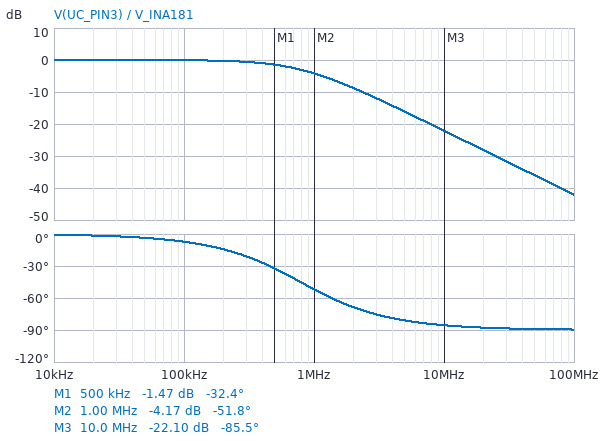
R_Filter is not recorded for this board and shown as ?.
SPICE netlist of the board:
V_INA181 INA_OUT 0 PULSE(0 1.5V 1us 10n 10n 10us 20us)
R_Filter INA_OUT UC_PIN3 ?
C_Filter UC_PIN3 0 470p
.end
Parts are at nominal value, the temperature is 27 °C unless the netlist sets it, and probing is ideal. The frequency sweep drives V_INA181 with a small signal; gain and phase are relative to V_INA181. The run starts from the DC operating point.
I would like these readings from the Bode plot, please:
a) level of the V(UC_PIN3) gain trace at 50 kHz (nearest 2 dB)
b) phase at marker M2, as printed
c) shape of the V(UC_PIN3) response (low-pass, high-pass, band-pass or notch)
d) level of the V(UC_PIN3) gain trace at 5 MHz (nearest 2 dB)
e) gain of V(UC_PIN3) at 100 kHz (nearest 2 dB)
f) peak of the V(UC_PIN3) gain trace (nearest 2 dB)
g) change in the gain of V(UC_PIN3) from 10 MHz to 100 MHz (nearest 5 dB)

0 dB
-51.8 deg
low-pass
-16 dB
0 dB
0 dB
-20 dB
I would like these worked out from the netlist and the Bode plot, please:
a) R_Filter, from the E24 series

430 Ω
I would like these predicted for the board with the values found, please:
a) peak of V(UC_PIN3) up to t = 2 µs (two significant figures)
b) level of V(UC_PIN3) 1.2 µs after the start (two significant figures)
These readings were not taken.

1.5 V
930 mV
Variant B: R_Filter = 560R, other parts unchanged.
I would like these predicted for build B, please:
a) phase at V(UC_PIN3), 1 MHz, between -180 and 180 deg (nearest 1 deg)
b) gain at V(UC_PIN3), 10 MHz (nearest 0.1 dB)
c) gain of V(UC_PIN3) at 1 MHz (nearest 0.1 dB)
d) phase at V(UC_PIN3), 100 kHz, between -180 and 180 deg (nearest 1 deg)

-59 deg
-24.4 dB
-5.7 dB
-9 deg
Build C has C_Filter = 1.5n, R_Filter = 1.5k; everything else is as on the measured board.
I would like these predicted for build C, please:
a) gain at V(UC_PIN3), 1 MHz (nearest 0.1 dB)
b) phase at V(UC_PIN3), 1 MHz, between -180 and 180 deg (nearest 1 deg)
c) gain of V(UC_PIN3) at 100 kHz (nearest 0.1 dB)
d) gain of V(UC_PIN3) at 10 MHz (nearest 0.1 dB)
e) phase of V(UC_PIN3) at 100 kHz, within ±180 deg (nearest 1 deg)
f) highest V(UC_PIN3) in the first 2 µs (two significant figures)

-23.0 dB
-86 deg
-4.8 dB
-43.0 dB
-55 deg
540 mV
